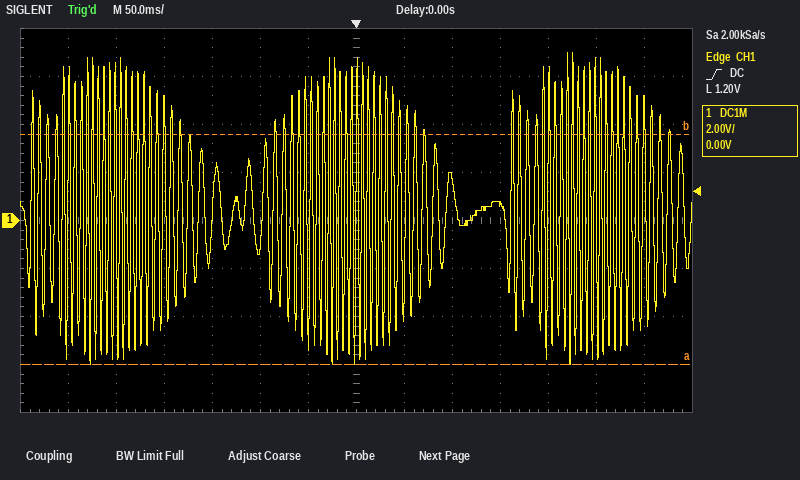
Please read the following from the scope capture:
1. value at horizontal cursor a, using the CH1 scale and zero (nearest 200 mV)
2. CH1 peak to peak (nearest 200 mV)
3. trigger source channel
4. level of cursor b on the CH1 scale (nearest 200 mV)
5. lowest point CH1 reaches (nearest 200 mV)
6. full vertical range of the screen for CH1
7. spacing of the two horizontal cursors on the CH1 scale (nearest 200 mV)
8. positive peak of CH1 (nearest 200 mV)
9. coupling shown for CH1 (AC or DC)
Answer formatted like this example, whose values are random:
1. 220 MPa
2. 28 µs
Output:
1. -6.0 V
2. 13.0 V
3. CH1
4. 3.6 V
5. -6.0 V
6. 16 V
7. 9.6 V
8. 7.0 V
9. DC
